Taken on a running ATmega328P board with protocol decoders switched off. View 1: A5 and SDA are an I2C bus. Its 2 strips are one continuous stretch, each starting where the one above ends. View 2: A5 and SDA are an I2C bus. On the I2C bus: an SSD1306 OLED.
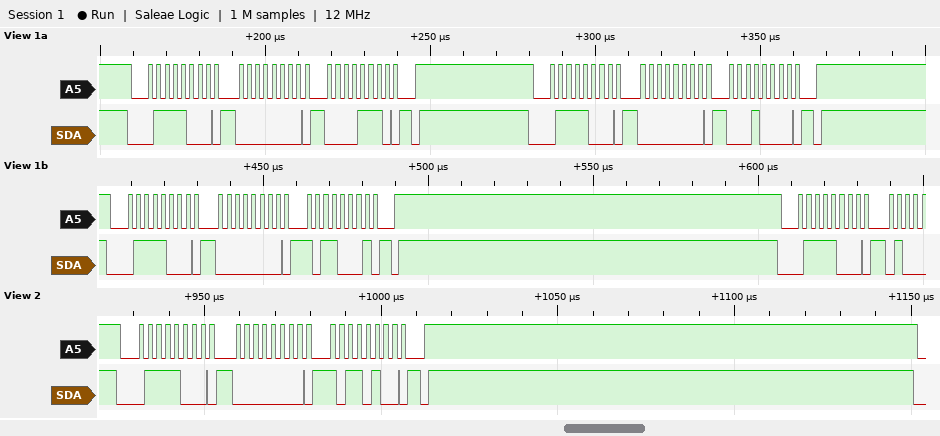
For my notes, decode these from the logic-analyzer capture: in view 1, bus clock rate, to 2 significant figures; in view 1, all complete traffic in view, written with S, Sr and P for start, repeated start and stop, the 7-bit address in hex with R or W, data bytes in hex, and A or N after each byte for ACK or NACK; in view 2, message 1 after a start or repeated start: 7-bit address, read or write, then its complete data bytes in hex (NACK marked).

400 kHz
S 3CW A 00 A 0E A P S 3CW A 00 A 10 A P S 3CW A 00 A B1 A P S 3CW A
0x3C write: 00 B4
